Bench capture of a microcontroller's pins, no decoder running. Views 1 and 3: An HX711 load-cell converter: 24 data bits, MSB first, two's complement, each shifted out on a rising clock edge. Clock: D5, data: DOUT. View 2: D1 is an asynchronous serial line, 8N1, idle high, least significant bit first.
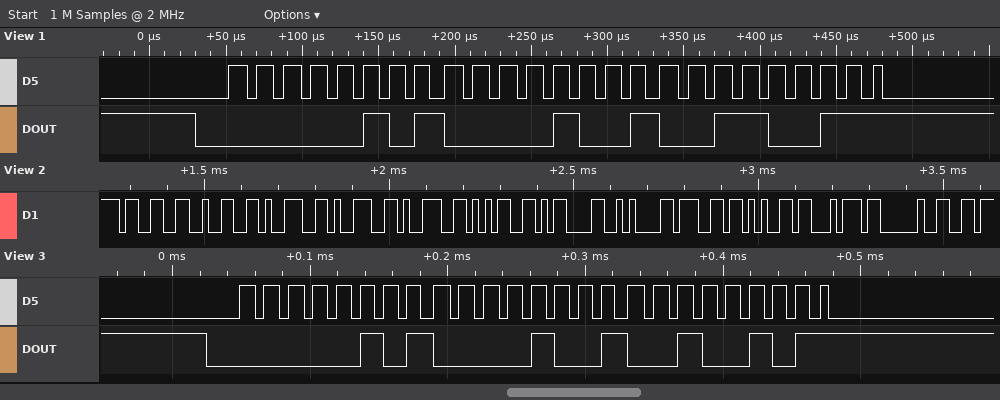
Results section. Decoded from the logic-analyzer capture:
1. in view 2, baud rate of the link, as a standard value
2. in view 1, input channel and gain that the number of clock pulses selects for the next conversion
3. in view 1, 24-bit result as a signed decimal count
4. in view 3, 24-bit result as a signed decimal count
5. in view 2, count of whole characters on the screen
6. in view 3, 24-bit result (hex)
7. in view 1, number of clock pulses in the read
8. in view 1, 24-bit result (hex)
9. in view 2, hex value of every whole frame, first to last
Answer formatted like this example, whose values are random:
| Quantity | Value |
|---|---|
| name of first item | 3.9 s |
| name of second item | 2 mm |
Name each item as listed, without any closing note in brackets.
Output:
| Quantity | Value |
|---|---|
| in view 2, baud rate of the link, as a standard value | 57600 baud |
| in view 1, input channel and gain that the number of clock pulses selects for the next conversion | channel A, gain 128 |
| in view 1, 24-bit result as a signed decimal count | 330035 |
| in view 3, 24-bit result as a signed decimal count | 330021 |
| in view 2, count of whole characters on the screen | 12 |
| in view 3, 24-bit result | 0x050925 |
| in view 1, number of clock pulses in the read | 25 |
| in view 1, 24-bit result | 0x050933 |
| in view 2, hex value of every whole frame, first to last | 33 32 39 39 39 35 0D 0A 67 65 74 20 |
